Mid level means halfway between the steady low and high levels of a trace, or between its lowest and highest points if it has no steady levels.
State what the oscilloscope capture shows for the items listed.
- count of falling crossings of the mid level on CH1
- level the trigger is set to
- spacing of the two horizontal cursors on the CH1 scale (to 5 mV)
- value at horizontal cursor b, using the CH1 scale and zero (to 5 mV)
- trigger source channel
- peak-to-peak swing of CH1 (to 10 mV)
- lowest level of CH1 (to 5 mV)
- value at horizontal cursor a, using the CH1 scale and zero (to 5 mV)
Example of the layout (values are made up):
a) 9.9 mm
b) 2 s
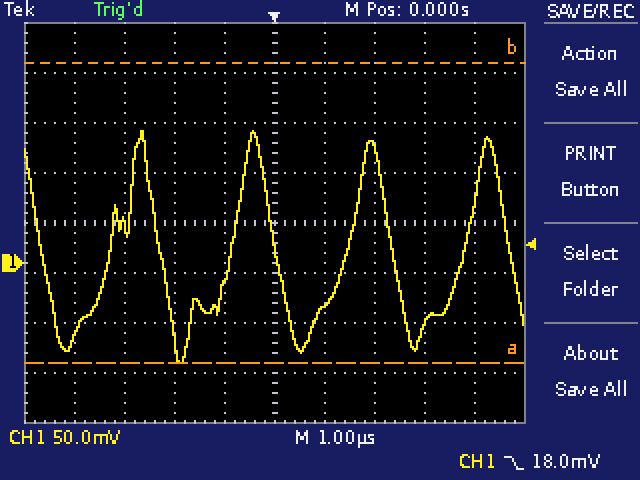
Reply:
a) 5
b) 18.0 mV
c) 300 mV
d) 200 mV
e) CH1
f) 230 mV
g) -100 mV
h) -100 mV
